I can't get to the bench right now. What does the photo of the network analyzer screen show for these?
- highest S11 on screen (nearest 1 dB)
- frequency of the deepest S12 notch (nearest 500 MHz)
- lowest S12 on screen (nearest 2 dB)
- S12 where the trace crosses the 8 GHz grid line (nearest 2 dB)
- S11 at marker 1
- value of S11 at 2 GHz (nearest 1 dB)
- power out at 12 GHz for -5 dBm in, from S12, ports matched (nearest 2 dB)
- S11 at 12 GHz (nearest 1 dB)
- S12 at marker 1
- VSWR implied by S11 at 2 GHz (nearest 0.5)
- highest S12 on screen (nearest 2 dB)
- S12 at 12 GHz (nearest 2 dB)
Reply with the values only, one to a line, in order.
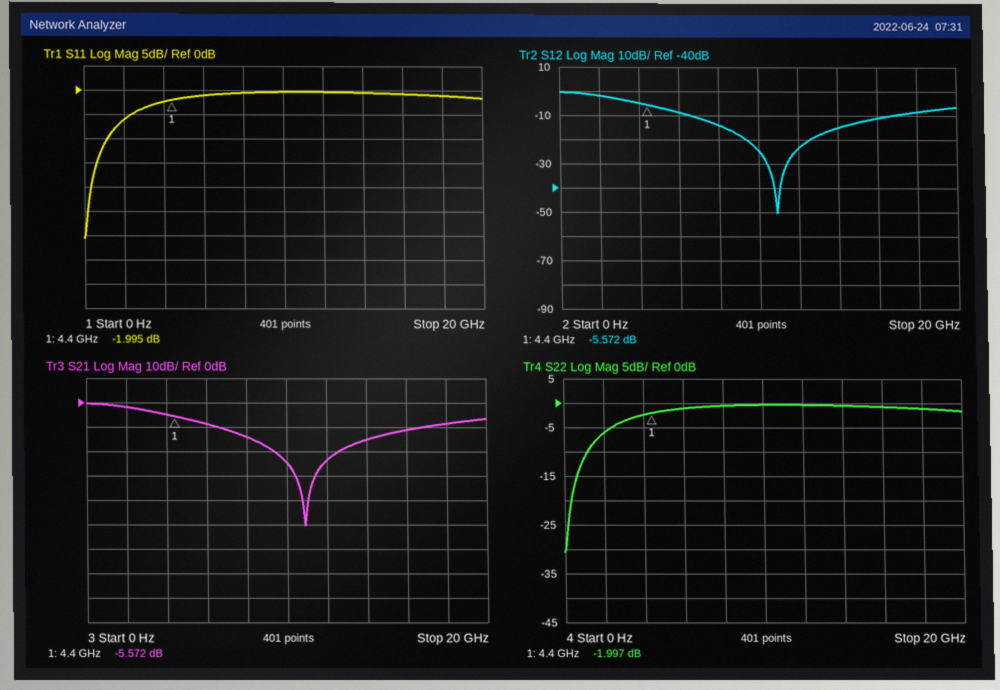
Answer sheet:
0 dB
11.0 GHz
-50 dB
-14 dB
-1.995 dB
-6 dB
-28 dBm
0 dB
-5.572 dB
3.0
0 dB
-24 dB
